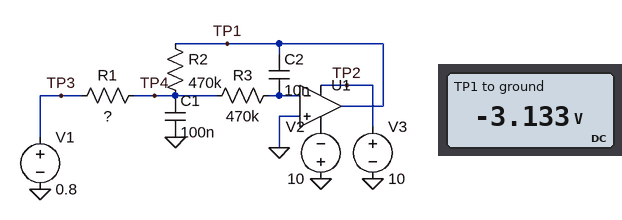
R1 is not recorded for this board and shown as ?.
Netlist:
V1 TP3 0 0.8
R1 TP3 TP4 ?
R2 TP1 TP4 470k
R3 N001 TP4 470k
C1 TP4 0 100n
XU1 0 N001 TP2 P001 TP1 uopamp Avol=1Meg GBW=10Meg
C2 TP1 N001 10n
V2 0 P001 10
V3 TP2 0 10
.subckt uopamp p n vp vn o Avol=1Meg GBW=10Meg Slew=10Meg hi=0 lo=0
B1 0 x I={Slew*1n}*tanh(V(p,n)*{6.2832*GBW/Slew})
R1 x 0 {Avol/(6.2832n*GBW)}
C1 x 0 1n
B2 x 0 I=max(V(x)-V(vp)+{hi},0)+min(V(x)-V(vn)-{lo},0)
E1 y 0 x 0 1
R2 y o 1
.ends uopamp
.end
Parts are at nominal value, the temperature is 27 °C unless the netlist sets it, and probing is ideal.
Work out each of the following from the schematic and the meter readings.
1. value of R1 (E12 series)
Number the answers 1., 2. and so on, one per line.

1. 120 kΩ
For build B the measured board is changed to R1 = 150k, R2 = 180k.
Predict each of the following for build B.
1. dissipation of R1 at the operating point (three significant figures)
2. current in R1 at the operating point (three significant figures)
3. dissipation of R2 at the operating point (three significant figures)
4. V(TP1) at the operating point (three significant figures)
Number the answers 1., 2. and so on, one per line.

1. 4.27 µW
2. 5.33 µA
3. 5.12 µW
4. -960 mV
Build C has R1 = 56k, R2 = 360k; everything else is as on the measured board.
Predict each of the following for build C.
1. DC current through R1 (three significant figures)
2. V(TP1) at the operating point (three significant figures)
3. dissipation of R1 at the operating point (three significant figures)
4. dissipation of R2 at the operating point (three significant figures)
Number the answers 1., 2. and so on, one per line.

1. 14.3 µA
2. -5.14 V
3. 11.4 µW
4. 73.5 µW
